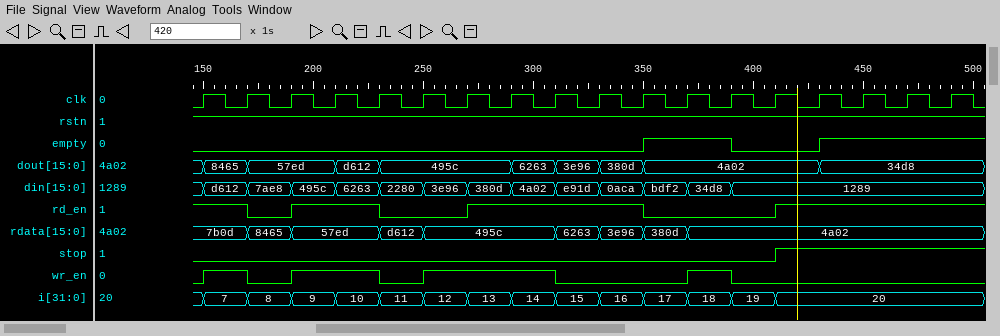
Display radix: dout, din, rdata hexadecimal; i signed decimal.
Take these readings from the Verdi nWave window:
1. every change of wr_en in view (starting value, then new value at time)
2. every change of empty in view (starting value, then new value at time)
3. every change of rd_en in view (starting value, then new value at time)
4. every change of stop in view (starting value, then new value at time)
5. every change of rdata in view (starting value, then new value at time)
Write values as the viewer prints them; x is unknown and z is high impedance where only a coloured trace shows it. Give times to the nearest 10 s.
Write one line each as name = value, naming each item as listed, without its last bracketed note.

every change of wr_en in view = 0, 1 at 150 s, 0 at 170 s, 1 at 190 s, 0 at 230 s, 1 at 250 s, 0 at 310 s, 1 at 370 s, 0 at 390 s
every change of empty in view = 0, 1 at 350 s, 0 at 390 s, 1 at 430 s
every change of rd_en in view = 1, 0 at 170 s, 1 at 190 s, 0 at 230 s, 1 at 270 s, 0 at 350 s, 1 at 410 s
every change of stop in view = 0, 1 at 410 s
every change of rdata in view = 7b0d, 8465 at 170 s, 57ed at 190 s, d612 at 230 s, 495c at 250 s, 6263 at 310 s, 3e96 at 330 s, 380d at 350 s, 4a02 at 370 s
